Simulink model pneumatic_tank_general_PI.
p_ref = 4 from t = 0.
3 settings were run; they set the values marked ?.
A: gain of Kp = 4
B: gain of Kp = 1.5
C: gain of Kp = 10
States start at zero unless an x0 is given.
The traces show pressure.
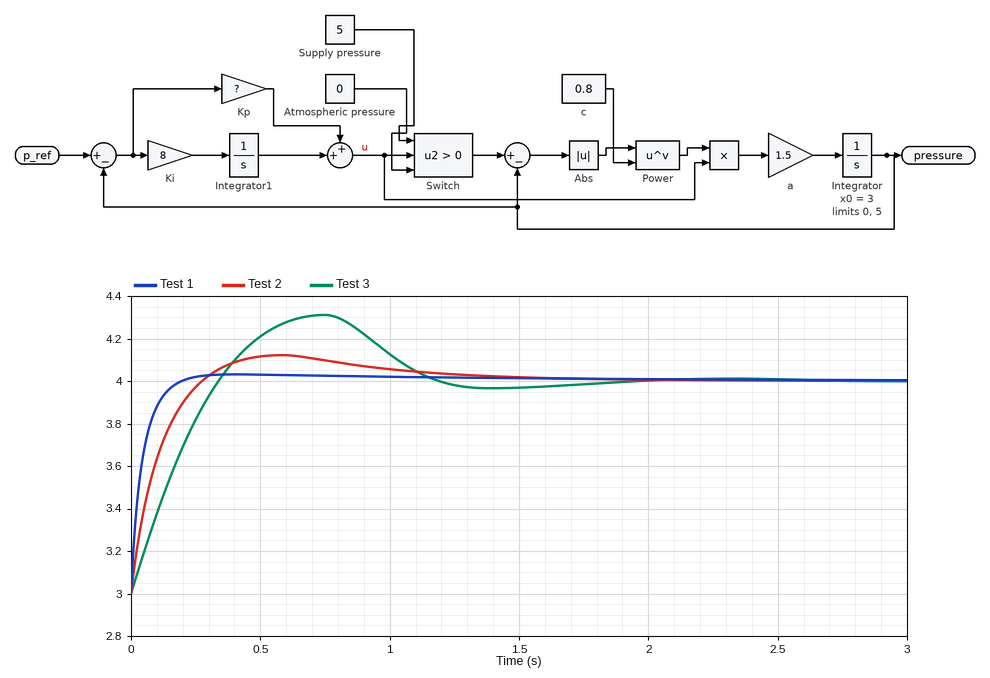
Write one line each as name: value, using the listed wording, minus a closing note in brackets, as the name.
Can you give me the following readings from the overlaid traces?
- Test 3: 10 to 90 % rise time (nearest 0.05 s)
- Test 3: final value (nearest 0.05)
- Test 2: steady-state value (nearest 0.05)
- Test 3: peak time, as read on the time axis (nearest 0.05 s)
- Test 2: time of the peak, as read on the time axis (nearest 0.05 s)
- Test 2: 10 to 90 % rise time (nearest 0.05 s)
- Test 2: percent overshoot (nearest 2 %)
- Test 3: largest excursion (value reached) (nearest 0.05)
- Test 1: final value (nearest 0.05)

Test 3: 10 to 90 % rise time: 0.25 s
Test 3: final value: 4.00
Test 2: steady-state value: 4.00
Test 3: peak time, as read on the time axis: 0.75 s
Test 2: time of the peak, as read on the time axis: 0.60 s
Test 2: 10 to 90 % rise time: 0.20 s
Test 2: percent overshoot: 12 %
Test 3: largest excursion (value reached): 4.30
Test 1: final value: 4.00
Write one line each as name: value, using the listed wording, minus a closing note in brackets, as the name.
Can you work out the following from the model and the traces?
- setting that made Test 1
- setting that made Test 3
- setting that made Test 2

setting that made Test 1: C
setting that made Test 3: B
setting that made Test 2: A
